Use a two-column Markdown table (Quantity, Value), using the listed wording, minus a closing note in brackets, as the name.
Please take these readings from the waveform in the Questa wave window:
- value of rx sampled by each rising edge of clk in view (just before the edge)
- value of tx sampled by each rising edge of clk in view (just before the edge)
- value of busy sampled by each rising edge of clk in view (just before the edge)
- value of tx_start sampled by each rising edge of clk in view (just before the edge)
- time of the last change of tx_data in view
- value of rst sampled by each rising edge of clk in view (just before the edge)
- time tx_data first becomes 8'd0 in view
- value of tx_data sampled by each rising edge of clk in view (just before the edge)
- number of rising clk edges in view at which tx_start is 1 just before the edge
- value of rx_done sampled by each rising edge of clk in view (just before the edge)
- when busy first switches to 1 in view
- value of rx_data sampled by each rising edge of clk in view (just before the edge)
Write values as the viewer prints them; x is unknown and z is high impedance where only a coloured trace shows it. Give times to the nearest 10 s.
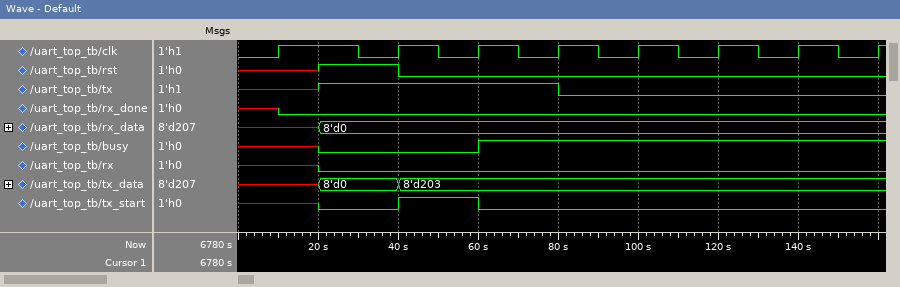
| Quantity | Value |
|---|---|
| value of rx sampled by each rising edge of clk in view | x 0 0 0 0 0 0 0 |
| value of tx sampled by each rising edge of clk in view | x 1 1 1 0 0 0 0 |
| value of busy sampled by each rising edge of clk in view | x 0 0 1 1 1 1 1 |
| value of tx_start sampled by each rising edge of clk in view | x 0 1 0 0 0 0 0 |
| time of the last change of tx_data in view | 40 s |
| value of rst sampled by each rising edge of clk in view | x 1 0 0 0 0 0 0 |
| time tx_data first becomes 8'd0 in view | 20 s |
| value of tx_data sampled by each rising edge of clk in view | x, 8'd0, 8'd203, 8'd203, 8'd203, 8'd203, 8'd203, 8'd203 |
| number of rising clk edges in view at which tx_start is 1 just before the edge | 1 |
| value of rx_done sampled by each rising edge of clk in view | x 0 0 0 0 0 0 0 |
| when busy first switches to 1 in view | 60 s |
| value of rx_data sampled by each rising edge of clk in view | x, 8'd0, 8'd0, 8'd0, 8'd0, 8'd0, 8'd0, 8'd0 |
